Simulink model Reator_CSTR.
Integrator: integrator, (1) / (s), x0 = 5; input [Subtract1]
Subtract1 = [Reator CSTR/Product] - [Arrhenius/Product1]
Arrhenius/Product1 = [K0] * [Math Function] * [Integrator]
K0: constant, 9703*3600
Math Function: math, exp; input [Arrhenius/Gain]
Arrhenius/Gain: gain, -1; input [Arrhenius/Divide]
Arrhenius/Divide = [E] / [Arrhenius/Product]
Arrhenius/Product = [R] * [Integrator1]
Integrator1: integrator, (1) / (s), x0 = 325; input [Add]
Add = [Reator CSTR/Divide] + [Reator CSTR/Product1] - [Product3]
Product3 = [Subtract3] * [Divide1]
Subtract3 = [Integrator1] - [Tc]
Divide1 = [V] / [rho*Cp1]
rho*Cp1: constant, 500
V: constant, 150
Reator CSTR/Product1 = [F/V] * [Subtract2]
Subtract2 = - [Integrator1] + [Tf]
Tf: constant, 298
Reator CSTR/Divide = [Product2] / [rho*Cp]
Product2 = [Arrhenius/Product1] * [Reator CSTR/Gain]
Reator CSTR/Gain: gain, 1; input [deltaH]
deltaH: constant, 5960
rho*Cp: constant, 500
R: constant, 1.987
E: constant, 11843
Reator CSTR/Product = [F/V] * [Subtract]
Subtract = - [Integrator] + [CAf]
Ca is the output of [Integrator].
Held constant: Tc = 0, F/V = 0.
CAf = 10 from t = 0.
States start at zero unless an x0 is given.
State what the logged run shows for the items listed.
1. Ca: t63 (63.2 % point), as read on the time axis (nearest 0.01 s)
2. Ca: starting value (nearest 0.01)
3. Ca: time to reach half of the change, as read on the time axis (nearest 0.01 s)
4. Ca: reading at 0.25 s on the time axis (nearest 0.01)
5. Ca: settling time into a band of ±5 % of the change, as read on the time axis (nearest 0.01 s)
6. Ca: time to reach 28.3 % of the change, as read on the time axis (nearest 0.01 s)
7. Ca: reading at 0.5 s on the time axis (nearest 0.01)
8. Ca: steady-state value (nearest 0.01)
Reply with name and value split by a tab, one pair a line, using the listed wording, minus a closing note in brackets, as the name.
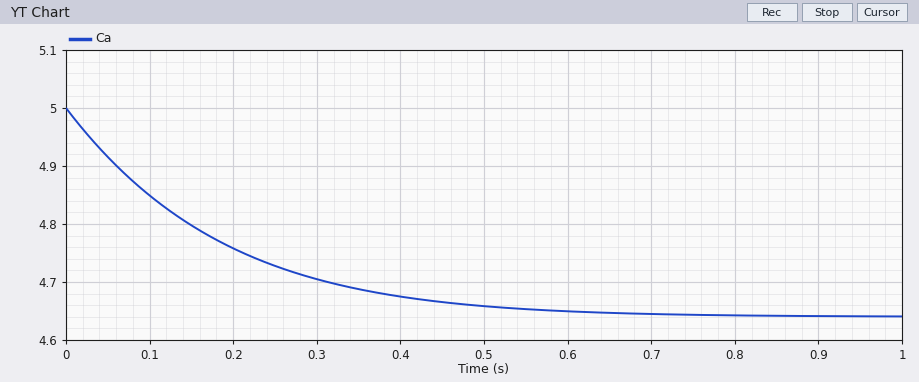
Ca: t63 (63.2 % point), as read on the time axis	0.18 s
Ca: starting value	5.00
Ca: time to reach half of the change, as read on the time axis	0.13 s
Ca: reading at 0.25 s on the time axis	4.73
Ca: settling time into a band of ±5 % of the change, as read on the time axis	0.50 s
Ca: time to reach 28.3 % of the change, as read on the time axis	0.06 s
Ca: reading at 0.5 s on the time axis	4.66
Ca: steady-state value	4.64
